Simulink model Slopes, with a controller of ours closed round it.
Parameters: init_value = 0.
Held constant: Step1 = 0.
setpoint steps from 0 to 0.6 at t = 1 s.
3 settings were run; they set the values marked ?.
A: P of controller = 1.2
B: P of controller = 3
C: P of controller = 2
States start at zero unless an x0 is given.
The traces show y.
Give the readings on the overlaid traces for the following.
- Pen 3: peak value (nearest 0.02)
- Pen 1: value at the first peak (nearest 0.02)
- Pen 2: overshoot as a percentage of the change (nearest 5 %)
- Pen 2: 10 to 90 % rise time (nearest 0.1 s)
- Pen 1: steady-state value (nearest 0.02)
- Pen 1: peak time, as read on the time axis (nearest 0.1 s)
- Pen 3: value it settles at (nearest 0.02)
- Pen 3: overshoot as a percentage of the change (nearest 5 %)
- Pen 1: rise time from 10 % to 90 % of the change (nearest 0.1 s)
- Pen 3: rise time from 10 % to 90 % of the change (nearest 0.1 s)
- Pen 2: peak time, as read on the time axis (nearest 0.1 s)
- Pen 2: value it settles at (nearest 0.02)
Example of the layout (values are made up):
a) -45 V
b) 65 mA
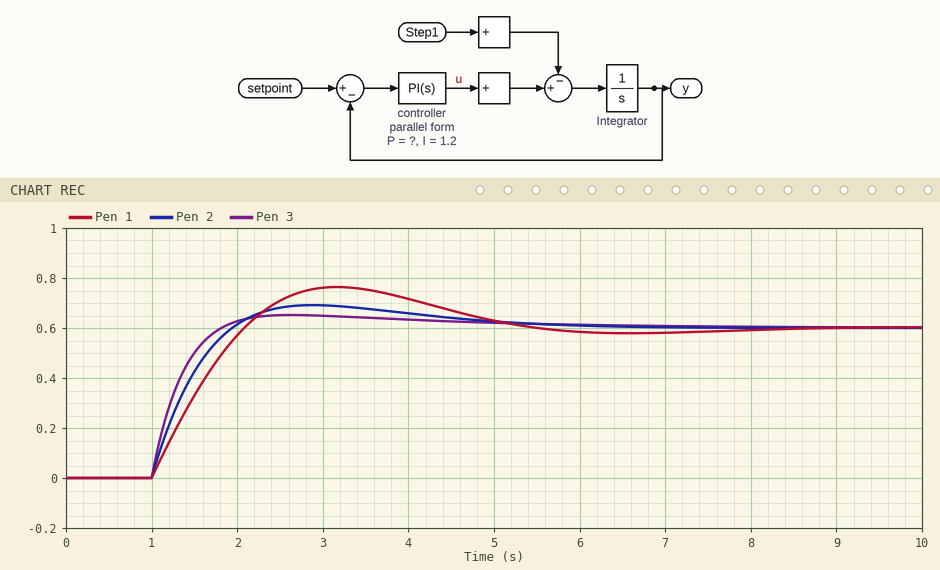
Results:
a) 0.66
b) 0.76
c) 15 %
d) 0.7 s
e) 0.60
f) 3.2 s
g) 0.60
h) 10 %
i) 0.8 s
j) 0.6 s
k) 2.9 s
l) 0.60
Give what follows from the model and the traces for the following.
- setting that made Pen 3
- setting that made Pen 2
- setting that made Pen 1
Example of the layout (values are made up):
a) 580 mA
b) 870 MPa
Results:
a) B
b) C
c) A
